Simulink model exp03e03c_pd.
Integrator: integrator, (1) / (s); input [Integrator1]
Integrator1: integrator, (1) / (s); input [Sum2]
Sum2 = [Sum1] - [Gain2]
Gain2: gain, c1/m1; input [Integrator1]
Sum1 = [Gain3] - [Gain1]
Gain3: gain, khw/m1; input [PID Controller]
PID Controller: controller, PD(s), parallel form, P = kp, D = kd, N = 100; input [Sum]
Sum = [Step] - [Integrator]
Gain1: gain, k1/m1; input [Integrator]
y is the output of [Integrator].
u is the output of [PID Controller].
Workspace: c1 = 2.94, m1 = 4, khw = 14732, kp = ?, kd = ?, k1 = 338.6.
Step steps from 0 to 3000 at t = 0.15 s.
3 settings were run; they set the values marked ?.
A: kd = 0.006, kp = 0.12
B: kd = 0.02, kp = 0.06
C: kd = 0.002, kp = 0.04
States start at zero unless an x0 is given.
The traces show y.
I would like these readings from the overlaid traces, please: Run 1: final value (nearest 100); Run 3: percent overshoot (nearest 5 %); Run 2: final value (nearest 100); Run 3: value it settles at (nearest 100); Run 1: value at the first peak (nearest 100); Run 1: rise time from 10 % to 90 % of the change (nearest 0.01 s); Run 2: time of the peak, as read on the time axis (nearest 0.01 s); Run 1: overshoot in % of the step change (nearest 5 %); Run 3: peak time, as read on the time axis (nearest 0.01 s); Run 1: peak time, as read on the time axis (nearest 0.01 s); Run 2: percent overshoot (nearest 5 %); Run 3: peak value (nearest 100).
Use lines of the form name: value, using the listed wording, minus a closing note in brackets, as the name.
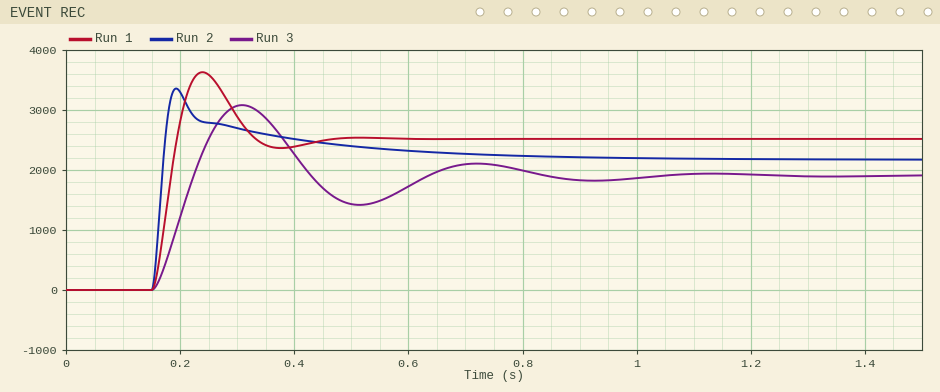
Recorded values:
Run 1: final value: 2500
Run 3: percent overshoot: 60 %
Run 2: final value: 2200
Run 3: value it settles at: 1900
Run 1: value at the first peak: 3600
Run 1: rise time from 10 % to 90 % of the change: 0.03 s
Run 2: time of the peak, as read on the time axis: 0.19 s
Run 1: overshoot in % of the step change: 45 %
Run 3: peak time, as read on the time axis: 0.31 s
Run 1: peak time, as read on the time axis: 0.24 s
Run 2: percent overshoot: 55 %
Run 3: peak value: 3100
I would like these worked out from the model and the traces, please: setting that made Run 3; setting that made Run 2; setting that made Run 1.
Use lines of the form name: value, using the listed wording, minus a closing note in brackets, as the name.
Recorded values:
setting that made Run 3: C
setting that made Run 2: B
setting that made Run 1: A
